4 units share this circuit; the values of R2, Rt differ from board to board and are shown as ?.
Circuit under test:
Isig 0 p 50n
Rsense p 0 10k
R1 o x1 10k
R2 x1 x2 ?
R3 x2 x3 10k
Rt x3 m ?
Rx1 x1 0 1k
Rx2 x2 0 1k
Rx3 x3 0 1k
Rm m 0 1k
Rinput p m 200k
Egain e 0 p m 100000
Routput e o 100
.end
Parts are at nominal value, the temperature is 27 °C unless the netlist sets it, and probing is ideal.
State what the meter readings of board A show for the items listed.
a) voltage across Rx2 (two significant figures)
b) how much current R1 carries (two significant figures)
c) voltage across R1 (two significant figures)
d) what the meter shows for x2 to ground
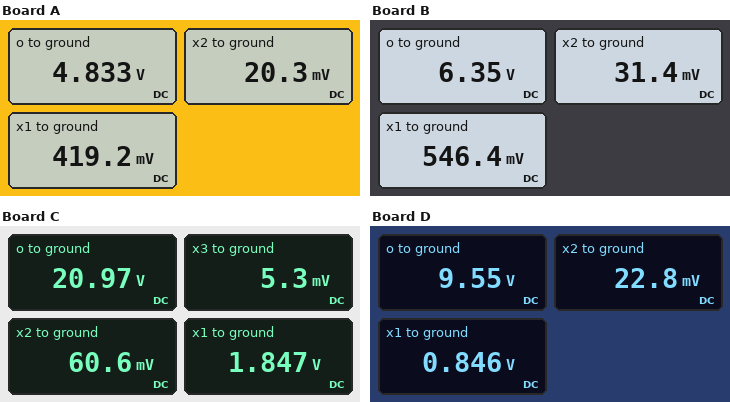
20 mV
440 µA
4.4 V
20.3 mV
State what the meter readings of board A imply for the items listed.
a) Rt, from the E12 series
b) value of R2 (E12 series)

2.2 kΩ
18 kΩ
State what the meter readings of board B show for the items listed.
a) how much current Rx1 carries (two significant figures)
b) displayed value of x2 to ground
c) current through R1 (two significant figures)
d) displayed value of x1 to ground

550 µA
31.4 mV
580 µA
546.4 mV
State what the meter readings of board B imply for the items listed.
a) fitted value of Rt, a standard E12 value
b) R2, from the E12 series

4.7 kΩ
15 kΩ
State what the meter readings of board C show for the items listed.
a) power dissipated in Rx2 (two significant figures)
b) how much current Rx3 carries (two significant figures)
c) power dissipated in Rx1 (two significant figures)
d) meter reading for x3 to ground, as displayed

3.7 µW
5.3 µA
3.4 mW
5.3 mV
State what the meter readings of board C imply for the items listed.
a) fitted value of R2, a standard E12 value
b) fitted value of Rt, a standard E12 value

27 kΩ
18 kΩ
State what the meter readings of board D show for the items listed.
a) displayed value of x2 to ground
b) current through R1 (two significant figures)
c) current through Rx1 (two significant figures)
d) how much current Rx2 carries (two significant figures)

22.8 mV
870 µA
850 µA
23 µA
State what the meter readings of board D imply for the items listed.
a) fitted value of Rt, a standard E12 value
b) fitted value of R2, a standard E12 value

3.3 kΩ
33 kΩ
